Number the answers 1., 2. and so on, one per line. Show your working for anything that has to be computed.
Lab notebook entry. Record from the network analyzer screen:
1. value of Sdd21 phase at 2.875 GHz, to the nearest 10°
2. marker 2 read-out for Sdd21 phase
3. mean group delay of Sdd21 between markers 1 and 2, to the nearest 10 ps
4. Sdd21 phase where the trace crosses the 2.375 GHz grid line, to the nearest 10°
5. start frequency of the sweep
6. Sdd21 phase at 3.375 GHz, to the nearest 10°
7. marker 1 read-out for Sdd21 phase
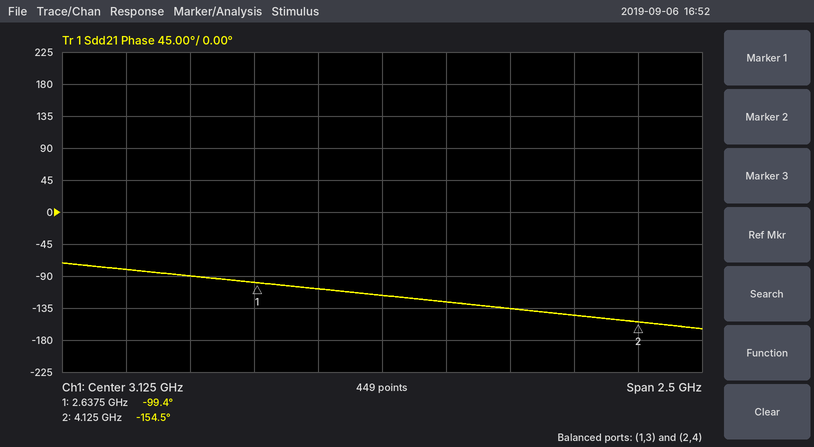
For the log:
1. -110°
2. -154.5°
3. −(-154.5° − (-99.4°))/(360° × 1.4875 GHz) ≈ 103 ps, so 100 ps to the nearest 10 ps
4. -90°
5. 1.875 GHz
6. -130°
7. -99.4°
